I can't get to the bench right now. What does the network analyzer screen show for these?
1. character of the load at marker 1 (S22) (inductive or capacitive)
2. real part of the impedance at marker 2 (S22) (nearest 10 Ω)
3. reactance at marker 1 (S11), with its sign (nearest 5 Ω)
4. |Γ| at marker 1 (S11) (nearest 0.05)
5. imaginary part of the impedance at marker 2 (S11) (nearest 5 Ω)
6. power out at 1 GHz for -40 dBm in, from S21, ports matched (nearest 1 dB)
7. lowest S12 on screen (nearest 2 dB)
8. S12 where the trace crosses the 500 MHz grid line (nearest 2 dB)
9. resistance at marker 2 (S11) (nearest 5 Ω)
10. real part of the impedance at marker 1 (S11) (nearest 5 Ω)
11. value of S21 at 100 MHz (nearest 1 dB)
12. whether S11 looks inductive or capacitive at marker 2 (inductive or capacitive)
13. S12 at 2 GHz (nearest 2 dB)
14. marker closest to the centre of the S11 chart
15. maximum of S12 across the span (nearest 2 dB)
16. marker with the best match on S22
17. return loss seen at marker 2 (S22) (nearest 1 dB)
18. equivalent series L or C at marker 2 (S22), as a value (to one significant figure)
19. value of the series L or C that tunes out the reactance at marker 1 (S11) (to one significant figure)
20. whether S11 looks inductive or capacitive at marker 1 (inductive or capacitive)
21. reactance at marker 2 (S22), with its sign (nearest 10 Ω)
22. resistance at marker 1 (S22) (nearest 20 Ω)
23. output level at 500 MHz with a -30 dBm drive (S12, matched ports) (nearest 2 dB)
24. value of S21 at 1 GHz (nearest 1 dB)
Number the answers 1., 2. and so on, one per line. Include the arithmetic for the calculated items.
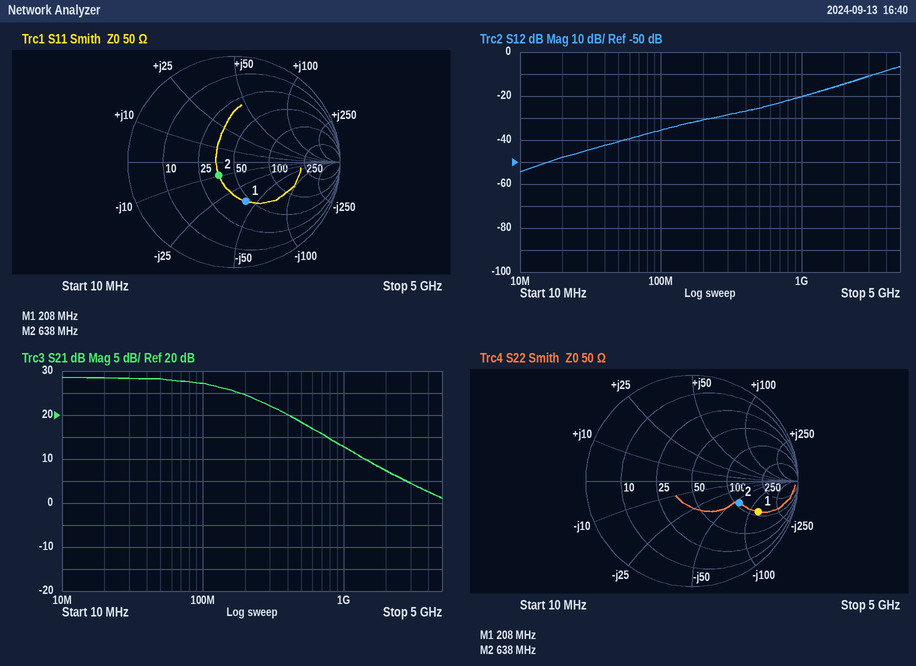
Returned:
1. capacitive
2. 110 Ω
3. -40 Ω
4. 0.40
5. -10 Ω
6. -40 dBm + (13 dB) = -27 dBm
7. -54 dB
8. -26 dB
9. 35 Ω
10. 45 Ω
11. 27 dB
12. capacitive
13. -14 dB
14. marker 2
15. -6 dB
16. marker 2
17. 6 dB
18. C = 1/(2π × 638 MHz × 60 Ω) ≈ 4 pF
19. L = 40 Ω/(2π × 208 MHz) ≈ 30.6 nH, so 30 nH to one significant figure
20. capacitive
21. -60 Ω
22. 120 Ω
23. -30 dBm + (-26 dB) = -56 dBm
24. 13 dB
